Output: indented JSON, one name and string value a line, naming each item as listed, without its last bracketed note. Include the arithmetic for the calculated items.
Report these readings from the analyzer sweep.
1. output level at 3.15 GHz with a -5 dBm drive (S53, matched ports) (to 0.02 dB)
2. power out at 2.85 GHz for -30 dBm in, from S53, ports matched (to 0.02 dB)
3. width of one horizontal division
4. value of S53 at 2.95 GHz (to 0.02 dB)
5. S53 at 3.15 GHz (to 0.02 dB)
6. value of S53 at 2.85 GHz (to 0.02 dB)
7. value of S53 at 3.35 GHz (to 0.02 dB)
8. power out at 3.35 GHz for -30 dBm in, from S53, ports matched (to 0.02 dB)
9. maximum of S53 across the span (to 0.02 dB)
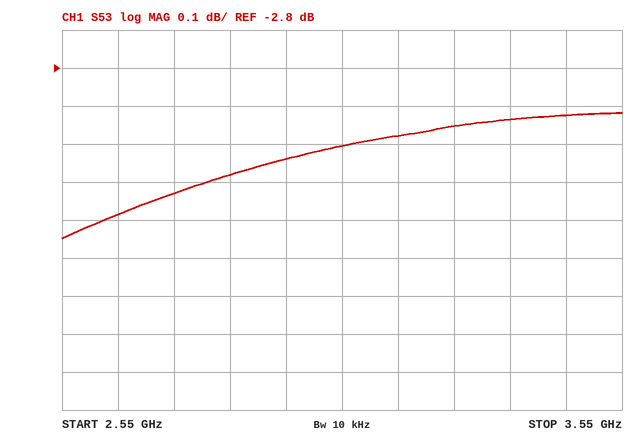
{
  "output level at 3.15 GHz with a -5 dBm drive (S53, matched ports)": "-5 dBm + (-2.98 dB) = -7.98 dBm",
  "power out at 2.85 GHz for -30 dBm in, from S53, ports matched": "-30 dBm + (-3.08 dB) = -33.08 dBm",
  "width of one horizontal division": "100 MHz",
  "value of S53 at 2.95 GHz": "-3.04 dB",
  "S53 at 3.15 GHz": "-2.98 dB",
  "value of S53 at 2.85 GHz": "-3.08 dB",
  "value of S53 at 3.35 GHz": "-2.94 dB",
  "power out at 3.35 GHz for -30 dBm in, from S53, ports matched": "-30 dBm + (-2.94 dB) = -32.94 dBm",
  "maximum of S53 across the span": "-2.92 dB"
}
